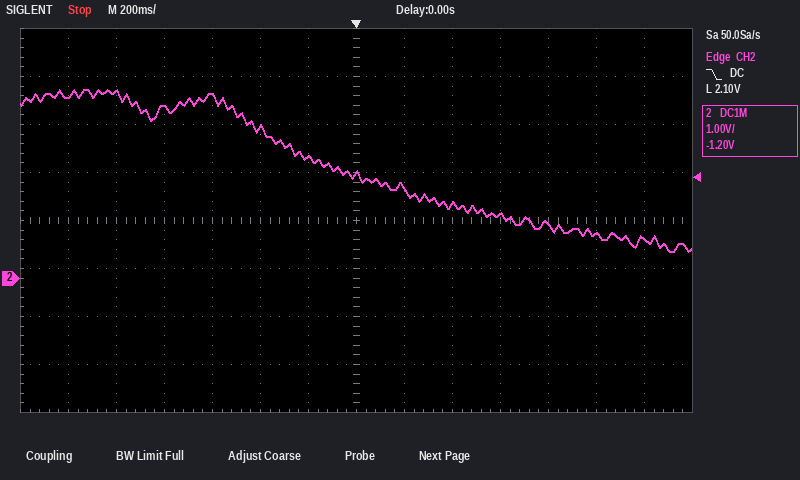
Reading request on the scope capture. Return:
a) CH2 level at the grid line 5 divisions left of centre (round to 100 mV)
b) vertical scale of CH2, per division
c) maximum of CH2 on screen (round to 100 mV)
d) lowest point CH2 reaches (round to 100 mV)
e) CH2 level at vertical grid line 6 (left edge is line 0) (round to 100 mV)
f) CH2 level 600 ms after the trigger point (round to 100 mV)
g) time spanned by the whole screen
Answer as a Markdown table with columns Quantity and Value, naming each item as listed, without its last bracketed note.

| Quantity | Value |
|---|---|
| CH2 level at the grid line 5 divisions left of centre | 3.9 V |
| vertical scale of CH2, per division | 1 V |
| maximum of CH2 on screen | 3.9 V |
| lowest point CH2 reaches | 600 mV |
| CH2 level at vertical grid line 6 (left edge is line 0) | 2.5 V |
| CH2 level 600 ms after the trigger point | 1.3 V |
| time spanned by the whole screen | 2.8 s |
